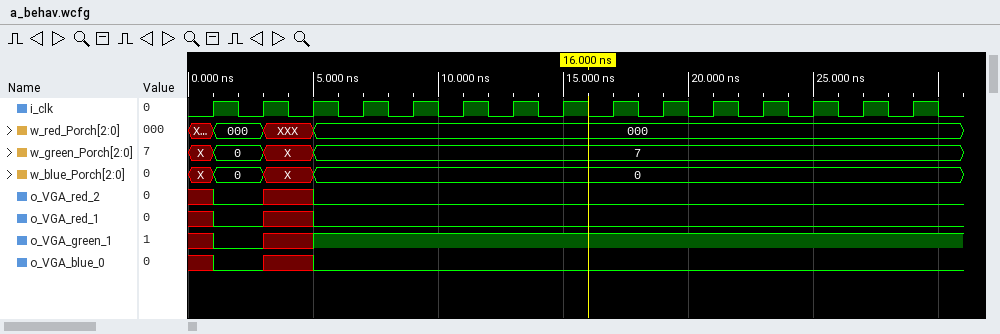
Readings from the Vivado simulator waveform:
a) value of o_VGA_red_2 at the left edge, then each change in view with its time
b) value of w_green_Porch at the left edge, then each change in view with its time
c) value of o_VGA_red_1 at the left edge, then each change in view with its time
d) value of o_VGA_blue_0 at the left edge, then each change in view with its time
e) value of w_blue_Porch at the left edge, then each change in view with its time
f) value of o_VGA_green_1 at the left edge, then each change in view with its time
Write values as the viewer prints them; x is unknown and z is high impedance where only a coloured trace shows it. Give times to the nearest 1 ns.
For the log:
x, 0 at 1 ns, x at 3 ns, 0 at 5 ns
X, 0 at 1 ns, X at 3 ns, 7 at 5 ns
x, 0 at 1 ns, x at 3 ns, 0 at 5 ns
x, 0 at 1 ns, x at 3 ns, 0 at 5 ns
X, 0 at 1 ns, X at 3 ns, 0 at 5 ns
x, 0 at 1 ns, x at 3 ns, 1 at 5 ns
